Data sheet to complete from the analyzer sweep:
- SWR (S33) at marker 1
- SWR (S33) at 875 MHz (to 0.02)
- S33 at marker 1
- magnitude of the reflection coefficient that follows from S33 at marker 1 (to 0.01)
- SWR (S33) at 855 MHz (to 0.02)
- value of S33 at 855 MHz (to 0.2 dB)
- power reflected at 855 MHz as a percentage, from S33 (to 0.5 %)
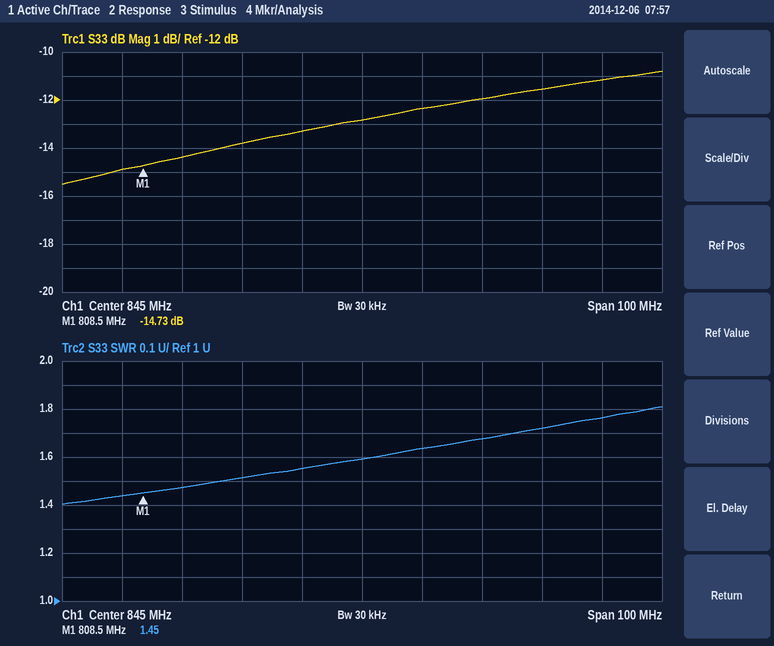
1.45
1.72
-14.73 dB
0.18
1.64
-12.4 dB
6.0 %
